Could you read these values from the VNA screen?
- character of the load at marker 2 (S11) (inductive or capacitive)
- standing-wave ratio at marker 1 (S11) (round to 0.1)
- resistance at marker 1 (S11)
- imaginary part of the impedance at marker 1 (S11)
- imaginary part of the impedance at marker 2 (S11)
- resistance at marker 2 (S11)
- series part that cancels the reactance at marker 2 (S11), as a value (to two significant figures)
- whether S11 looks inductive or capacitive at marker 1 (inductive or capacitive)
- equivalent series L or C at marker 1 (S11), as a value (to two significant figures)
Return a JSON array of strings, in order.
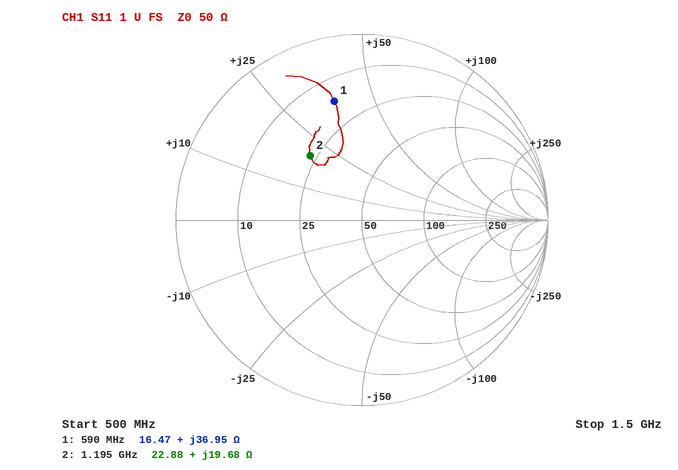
["inductive", "4.8", "16.47 Ω", "+36.95 Ω", "+19.68 Ω", "22.88 Ω", "6.8 pF", "inductive", "10.0 nH"]
